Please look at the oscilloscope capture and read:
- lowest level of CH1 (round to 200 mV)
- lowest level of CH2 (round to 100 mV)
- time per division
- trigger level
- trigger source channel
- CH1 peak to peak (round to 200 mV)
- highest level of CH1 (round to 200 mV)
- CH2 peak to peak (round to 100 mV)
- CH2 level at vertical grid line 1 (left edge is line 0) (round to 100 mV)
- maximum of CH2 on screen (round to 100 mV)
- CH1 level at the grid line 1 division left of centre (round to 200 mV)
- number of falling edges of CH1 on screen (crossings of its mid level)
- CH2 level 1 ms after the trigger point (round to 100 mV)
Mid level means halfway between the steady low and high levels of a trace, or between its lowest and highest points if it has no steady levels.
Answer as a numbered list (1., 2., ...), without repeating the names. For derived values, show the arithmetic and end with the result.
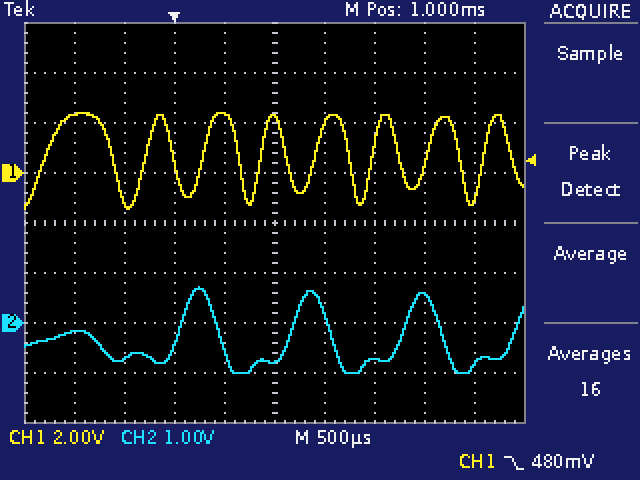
1. -1.4 V
2. -1.0 V
3. 500 µs
4. 480 mV
5. CH1
6. 2.4 V − (-1.4 V) = 3.8 V
7. 2.4 V
8. 700 mV − (-1.0 V) = 1.7 V
9. -200 mV
10. 700 mV
11. 2.4 V
12. 8
13. -800 mV
